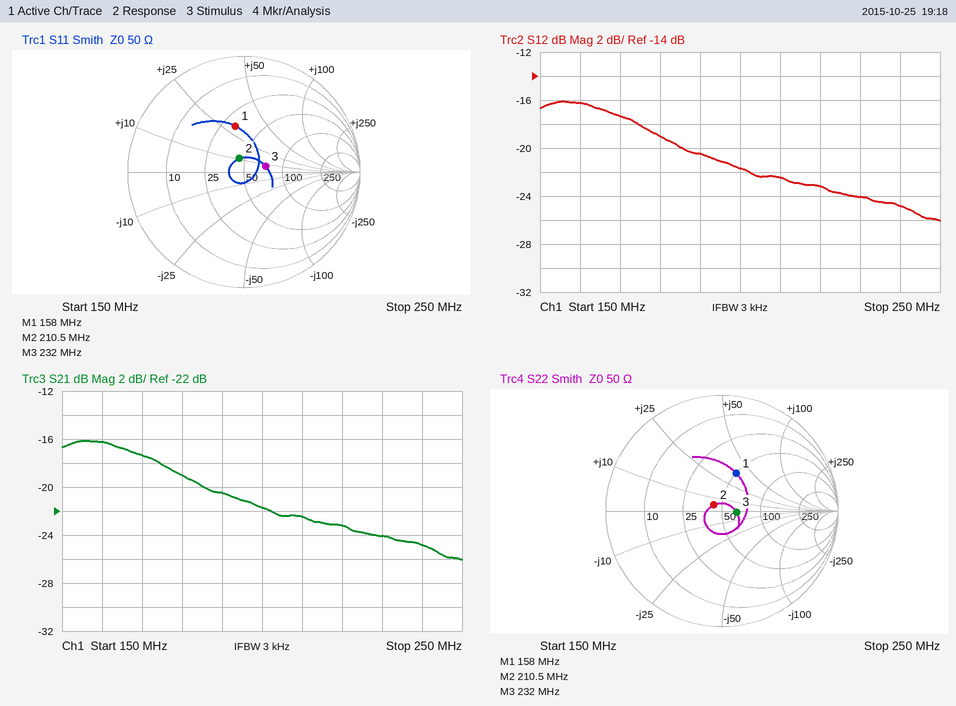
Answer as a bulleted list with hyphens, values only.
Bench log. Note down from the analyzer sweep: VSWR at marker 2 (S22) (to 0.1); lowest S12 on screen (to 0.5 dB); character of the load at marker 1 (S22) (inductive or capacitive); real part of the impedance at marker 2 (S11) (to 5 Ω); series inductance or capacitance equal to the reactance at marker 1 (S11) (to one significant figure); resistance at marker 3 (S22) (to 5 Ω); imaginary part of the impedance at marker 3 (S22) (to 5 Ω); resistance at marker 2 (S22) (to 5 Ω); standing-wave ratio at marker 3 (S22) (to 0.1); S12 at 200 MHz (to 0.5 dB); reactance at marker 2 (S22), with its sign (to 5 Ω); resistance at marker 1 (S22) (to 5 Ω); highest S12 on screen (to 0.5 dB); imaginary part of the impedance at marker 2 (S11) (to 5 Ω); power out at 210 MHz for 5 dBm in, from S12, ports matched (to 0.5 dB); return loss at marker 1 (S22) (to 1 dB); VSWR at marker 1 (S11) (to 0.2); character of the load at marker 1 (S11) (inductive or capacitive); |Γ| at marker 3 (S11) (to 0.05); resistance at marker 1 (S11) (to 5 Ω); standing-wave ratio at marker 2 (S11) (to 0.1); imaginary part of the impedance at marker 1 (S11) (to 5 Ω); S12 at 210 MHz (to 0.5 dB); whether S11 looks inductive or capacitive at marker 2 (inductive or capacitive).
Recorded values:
- 1.2
- -26.0 dB
- inductive
- 45 Ω
- 30 nH
- 65 Ω
- 0 Ω
- 45 Ω
- 1.3
- -21.5 dB
- +5 Ω
- 50 Ω
- -16.0 dB
- +10 Ω
- -17.5 dBm
- 9 dB
- 2.4
- inductive
- 0.20
- 30 Ω
- 1.3
- +30 Ω
- -22.5 dB
- inductive
